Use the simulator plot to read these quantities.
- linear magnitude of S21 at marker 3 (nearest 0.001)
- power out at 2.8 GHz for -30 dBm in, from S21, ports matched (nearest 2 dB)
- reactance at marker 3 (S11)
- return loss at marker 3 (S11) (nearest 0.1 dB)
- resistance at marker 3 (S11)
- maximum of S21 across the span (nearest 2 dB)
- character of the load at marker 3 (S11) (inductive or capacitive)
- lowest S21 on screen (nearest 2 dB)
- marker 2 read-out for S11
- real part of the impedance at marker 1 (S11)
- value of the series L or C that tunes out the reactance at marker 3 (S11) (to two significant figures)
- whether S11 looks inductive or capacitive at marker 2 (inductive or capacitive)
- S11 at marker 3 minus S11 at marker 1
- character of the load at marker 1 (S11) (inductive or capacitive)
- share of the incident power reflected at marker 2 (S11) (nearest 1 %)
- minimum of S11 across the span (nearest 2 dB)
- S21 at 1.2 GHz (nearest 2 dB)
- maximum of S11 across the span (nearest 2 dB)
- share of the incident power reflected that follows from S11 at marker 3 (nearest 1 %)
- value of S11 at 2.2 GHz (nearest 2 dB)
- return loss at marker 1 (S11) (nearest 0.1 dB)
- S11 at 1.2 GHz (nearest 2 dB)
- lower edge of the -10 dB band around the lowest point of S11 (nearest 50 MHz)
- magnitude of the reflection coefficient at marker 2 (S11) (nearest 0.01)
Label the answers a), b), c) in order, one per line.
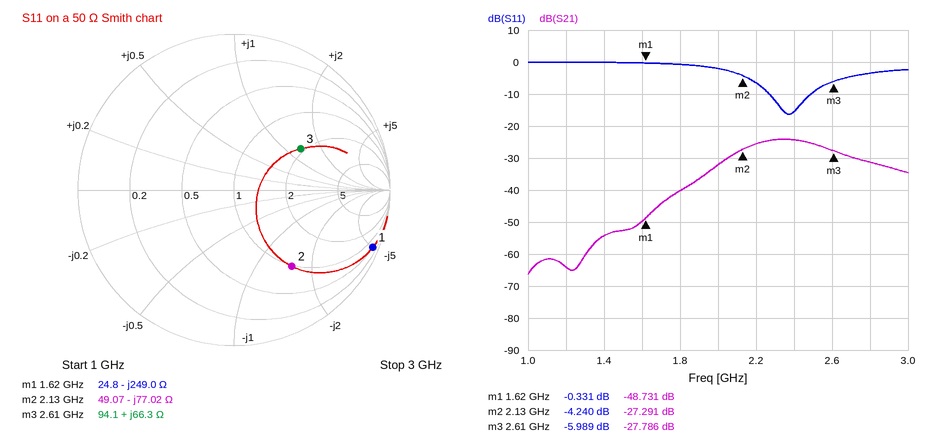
a) 0.041
b) -62 dBm
c) +66.3 Ω
d) 6.0 dB
e) 94.1 Ω
f) -24 dB
g) inductive
h) -66 dB
i) -4.240 dB
j) 24.8 Ω
k) 920 fF
l) capacitive
m) -5.658 dB
n) capacitive
o) 38 %
p) -16 dB
q) -64 dB
r) 0 dB
s) 25 %
t) -6 dB
u) 0.3 dB
v) 0 dB
w) 2.25 GHz
x) 0.61
